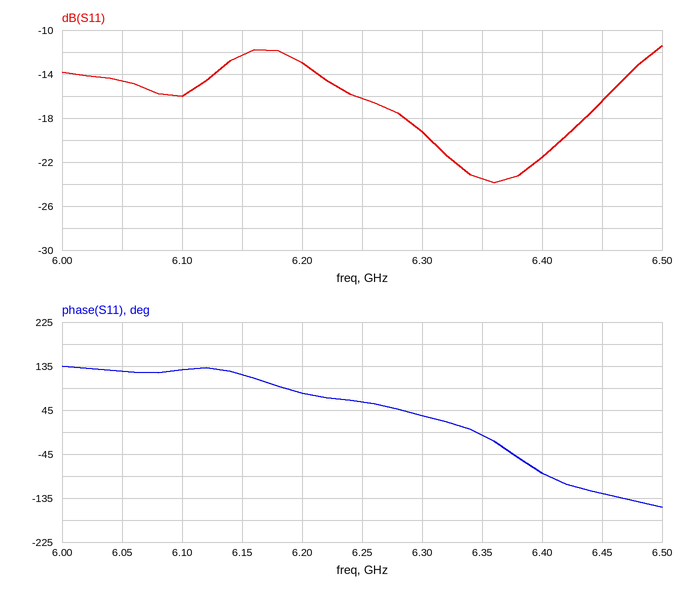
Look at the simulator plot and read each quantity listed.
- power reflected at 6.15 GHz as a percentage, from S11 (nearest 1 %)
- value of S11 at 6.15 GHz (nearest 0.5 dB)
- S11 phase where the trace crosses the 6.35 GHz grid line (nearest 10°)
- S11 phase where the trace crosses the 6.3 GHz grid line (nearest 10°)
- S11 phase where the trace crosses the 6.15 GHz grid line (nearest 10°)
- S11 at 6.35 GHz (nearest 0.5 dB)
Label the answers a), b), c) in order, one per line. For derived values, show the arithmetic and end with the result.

a) 10^(-12.5/10) ≈ 6 %
b) -12.5 dB
c) -10°
d) 30°
e) 120°
f) -23.5 dB
